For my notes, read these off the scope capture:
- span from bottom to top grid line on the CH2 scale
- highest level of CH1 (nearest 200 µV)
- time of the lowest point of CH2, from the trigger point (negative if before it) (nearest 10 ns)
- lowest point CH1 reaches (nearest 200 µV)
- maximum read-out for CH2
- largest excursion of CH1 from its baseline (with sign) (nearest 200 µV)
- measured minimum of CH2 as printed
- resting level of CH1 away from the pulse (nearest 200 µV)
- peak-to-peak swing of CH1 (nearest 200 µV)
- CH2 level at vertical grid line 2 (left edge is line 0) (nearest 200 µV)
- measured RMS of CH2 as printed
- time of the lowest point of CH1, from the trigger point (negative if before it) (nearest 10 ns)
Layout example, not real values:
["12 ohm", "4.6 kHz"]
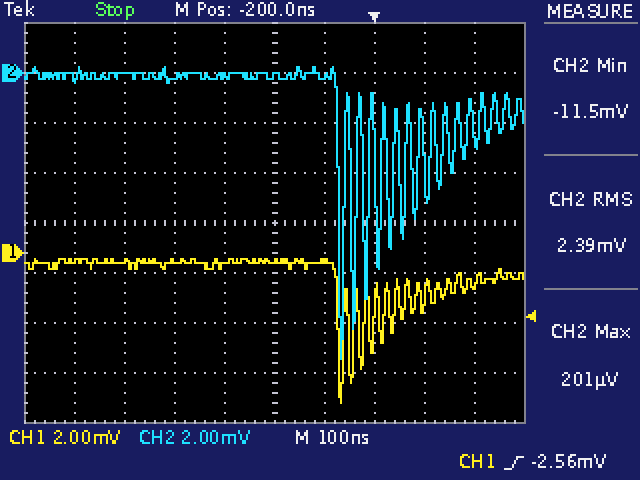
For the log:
["16 mV", "-200 µV", "-70 ns", "-6.0 mV", "201 µV", "-5.6 mV", "-11.5 mV", "-400 µV", "5.8 mV", "0.0 mV", "2.39 mV", "-70 ns"]
